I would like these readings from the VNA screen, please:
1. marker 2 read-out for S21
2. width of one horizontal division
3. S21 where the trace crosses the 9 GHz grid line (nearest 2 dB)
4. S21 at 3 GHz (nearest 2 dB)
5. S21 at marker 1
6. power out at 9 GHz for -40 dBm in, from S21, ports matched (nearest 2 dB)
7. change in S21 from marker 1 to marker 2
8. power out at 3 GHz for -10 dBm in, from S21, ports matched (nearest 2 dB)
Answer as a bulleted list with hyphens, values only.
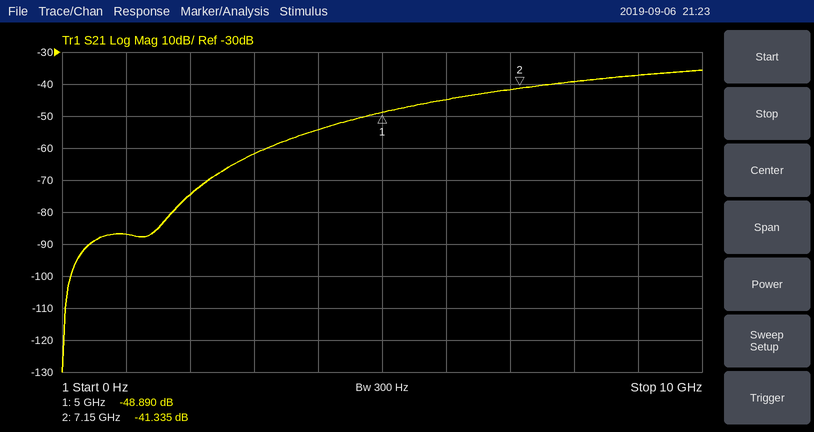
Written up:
- -41.335 dB
- 1 GHz
- -38 dB
- -62 dB
- -48.890 dB
- -78 dBm
- 7.555 dB
- -72 dBm
